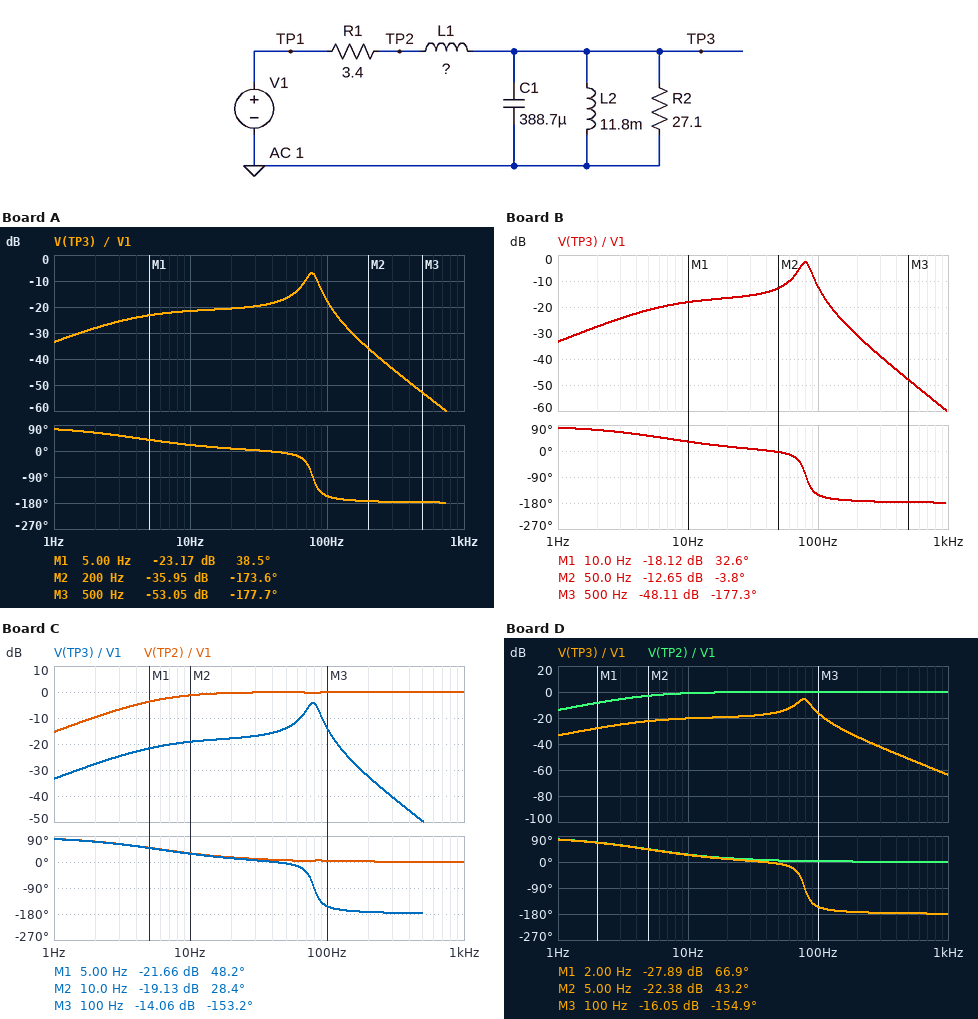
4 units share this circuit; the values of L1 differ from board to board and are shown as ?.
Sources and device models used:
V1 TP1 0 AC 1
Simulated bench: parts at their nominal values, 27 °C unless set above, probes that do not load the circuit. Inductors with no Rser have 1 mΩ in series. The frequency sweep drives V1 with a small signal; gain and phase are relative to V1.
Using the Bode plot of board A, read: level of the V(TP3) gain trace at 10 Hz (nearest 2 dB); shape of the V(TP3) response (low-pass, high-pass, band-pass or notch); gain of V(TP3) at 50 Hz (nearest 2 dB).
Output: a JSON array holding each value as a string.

["-22 dB", "band-pass", "-16 dB"]
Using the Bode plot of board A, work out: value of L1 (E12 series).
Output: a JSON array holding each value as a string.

["120 mH"]
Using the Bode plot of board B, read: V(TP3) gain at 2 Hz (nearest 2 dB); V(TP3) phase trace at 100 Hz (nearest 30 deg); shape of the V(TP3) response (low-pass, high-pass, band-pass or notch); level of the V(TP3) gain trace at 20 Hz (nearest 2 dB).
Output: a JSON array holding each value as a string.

["-28 dB", "-150 deg", "band-pass", "-16 dB"]
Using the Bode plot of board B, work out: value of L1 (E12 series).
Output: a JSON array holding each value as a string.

["68 mH"]
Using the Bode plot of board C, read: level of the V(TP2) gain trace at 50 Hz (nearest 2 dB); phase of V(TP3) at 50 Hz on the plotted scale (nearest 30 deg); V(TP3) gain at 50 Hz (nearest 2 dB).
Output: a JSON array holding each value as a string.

["0 dB", "0 deg", "-14 dB"]
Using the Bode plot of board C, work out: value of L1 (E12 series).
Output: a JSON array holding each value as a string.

["82 mH"]
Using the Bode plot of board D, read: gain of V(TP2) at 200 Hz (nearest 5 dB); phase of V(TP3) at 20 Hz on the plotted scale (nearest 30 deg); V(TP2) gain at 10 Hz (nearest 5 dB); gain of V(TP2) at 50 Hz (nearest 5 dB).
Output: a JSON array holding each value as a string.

["0 dB", "0 deg", "0 dB", "0 dB"]
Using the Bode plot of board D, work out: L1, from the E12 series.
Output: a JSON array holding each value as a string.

["100 mH"]
